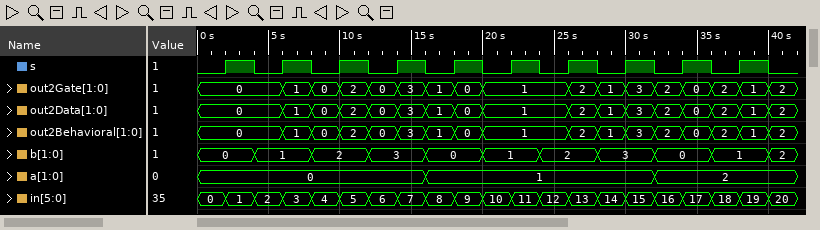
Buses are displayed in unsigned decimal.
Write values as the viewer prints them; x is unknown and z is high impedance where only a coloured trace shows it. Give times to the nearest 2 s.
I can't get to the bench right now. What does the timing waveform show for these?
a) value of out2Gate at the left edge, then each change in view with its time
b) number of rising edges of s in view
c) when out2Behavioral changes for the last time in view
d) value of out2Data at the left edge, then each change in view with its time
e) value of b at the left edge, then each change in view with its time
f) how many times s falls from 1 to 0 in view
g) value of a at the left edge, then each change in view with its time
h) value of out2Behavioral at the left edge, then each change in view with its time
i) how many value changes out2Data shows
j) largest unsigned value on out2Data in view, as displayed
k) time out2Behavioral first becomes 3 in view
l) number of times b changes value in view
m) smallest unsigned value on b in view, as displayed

0, 1 at 6 s, 0 at 8 s, 2 at 10 s, 0 at 12 s, 3 at 14 s, 1 at 16 s, 0 at 18 s, 1 at 20 s, 2 at 26 s, 1 at 28 s, 3 at 30 s, 2 at 32 s, 0 at 34 s, 2 at 36 s, 1 at 38 s, 2 at 40 s
10
40 s
0, 1 at 6 s, 0 at 8 s, 2 at 10 s, 0 at 12 s, 3 at 14 s, 1 at 16 s, 0 at 18 s, 1 at 20 s, 2 at 26 s, 1 at 28 s, 3 at 30 s, 2 at 32 s, 0 at 34 s, 2 at 36 s, 1 at 38 s, 2 at 40 s
0, 1 at 4 s, 2 at 8 s, 3 at 12 s, 0 at 16 s, 1 at 20 s, 2 at 24 s, 3 at 28 s, 0 at 32 s, 1 at 36 s, 2 at 40 s
10
0, 1 at 16 s, 2 at 32 s
0, 1 at 6 s, 0 at 8 s, 2 at 10 s, 0 at 12 s, 3 at 14 s, 1 at 16 s, 0 at 18 s, 1 at 20 s, 2 at 26 s, 1 at 28 s, 3 at 30 s, 2 at 32 s, 0 at 34 s, 2 at 36 s, 1 at 38 s, 2 at 40 s
16
3
14 s
10
0
